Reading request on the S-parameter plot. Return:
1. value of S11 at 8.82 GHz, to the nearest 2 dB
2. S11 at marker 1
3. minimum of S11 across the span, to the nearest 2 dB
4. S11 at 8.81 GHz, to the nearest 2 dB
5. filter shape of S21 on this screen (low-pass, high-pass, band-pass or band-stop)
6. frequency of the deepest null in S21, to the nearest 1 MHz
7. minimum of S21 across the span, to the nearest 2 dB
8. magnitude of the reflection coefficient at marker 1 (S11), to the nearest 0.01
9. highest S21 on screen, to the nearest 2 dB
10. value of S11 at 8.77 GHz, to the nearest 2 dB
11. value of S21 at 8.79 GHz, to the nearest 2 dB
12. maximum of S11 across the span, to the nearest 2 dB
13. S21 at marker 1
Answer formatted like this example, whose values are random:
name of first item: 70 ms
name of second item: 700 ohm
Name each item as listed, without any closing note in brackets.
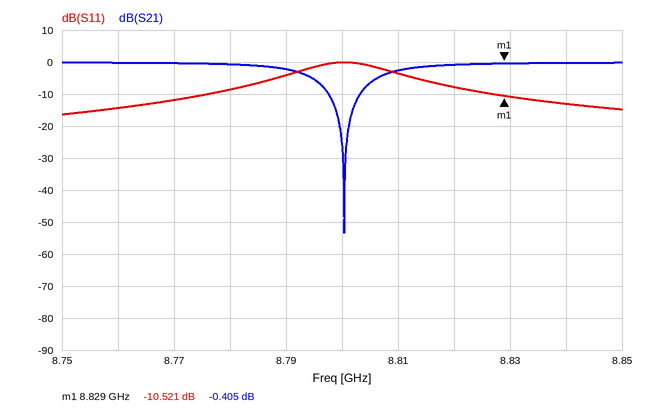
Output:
value of S11 at 8.82 GHz, to the nearest 2 dB: -8 dB
S11 at marker 1: -10.521 dB
minimum of S11 across the span, to the nearest 2 dB: -16 dB
S11 at 8.81 GHz, to the nearest 2 dB: -4 dB
filter shape of S21 on this screen: band-stop
frequency of the deepest null in S21, to the nearest 1 MHz: 8.800 GHz
minimum of S21 across the span, to the nearest 2 dB: -54 dB
magnitude of the reflection coefficient at marker 1 (S11), to the nearest 0.01: 0.30
highest S21 on screen, to the nearest 2 dB: 0 dB
value of S11 at 8.77 GHz, to the nearest 2 dB: -12 dB
value of S21 at 8.79 GHz, to the nearest 2 dB: -2 dB
maximum of S11 across the span, to the nearest 2 dB: 0 dB
S21 at marker 1: -0.405 dB
